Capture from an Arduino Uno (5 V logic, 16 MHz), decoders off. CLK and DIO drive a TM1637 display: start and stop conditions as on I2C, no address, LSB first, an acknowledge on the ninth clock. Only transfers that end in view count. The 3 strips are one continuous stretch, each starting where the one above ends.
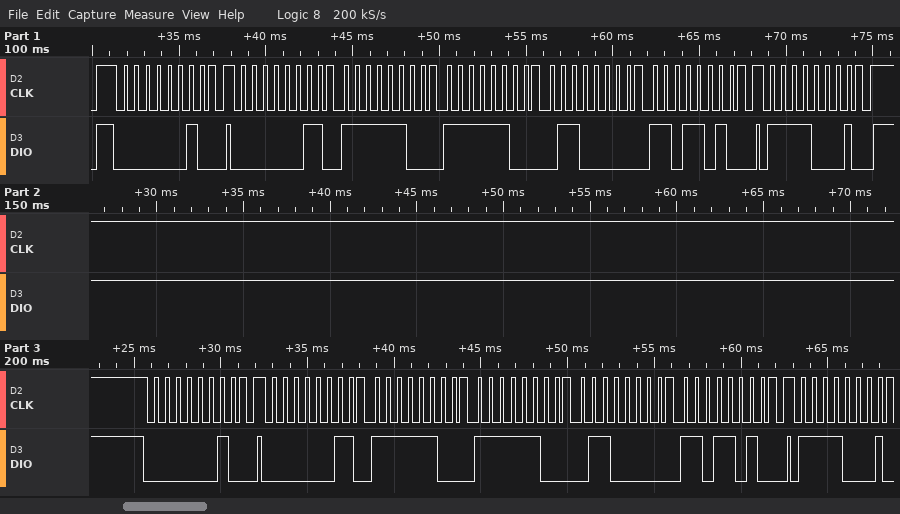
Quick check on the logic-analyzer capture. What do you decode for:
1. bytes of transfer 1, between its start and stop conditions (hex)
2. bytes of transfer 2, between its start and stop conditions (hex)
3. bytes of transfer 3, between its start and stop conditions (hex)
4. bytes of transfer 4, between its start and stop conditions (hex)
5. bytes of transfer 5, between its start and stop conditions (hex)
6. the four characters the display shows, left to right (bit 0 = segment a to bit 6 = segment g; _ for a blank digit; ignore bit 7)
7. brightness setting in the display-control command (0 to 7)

40
C0 3F 3F 06 5B
8F
40
C0 3F 3F 06 5B
0012
7
